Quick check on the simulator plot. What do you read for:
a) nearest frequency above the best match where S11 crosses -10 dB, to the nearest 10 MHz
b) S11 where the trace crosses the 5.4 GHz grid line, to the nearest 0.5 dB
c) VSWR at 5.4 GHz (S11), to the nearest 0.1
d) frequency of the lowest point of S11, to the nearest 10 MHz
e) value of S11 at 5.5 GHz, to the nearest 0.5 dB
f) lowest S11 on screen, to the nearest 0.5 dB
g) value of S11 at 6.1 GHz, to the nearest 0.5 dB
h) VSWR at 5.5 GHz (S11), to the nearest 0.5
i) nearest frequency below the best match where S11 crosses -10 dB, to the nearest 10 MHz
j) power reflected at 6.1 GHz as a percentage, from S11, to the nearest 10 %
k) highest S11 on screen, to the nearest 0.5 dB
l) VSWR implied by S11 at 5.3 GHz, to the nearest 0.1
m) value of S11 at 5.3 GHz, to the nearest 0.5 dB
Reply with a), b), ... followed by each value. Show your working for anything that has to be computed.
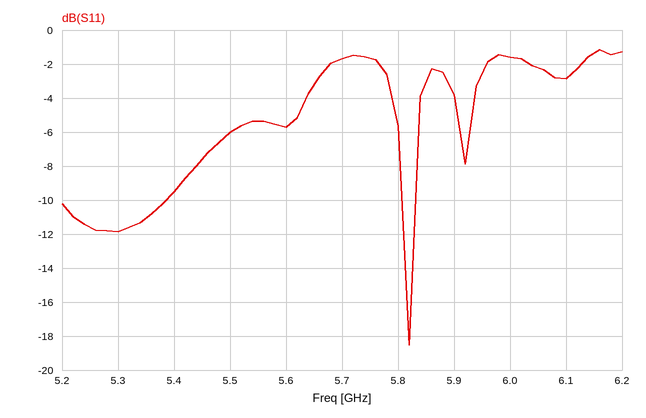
a) 5.83 GHz
b) -9.5 dB
c) |Γ| = 10^(-9.5/20) = 0.3350; VSWR = (1 + 0.3350)/(1 − 0.3350) ≈ 2.0
d) 5.82 GHz
e) -6.0 dB
f) -18.5 dB
g) -3.0 dB
h) |Γ| = 10^(-6/20) = 0.5012; VSWR = (1 + 0.5012)/(1 − 0.5012) ≈ 3.0
i) 5.81 GHz
j) 10^(-3/10) ≈ 50 %
k) -1.0 dB
l) |Γ| = 10^(-12/20) = 0.2512; VSWR = (1 + 0.2512)/(1 − 0.2512) ≈ 1.7
m) -12.0 dB
